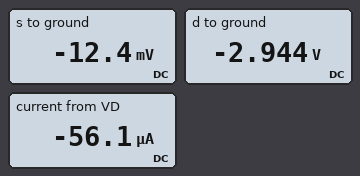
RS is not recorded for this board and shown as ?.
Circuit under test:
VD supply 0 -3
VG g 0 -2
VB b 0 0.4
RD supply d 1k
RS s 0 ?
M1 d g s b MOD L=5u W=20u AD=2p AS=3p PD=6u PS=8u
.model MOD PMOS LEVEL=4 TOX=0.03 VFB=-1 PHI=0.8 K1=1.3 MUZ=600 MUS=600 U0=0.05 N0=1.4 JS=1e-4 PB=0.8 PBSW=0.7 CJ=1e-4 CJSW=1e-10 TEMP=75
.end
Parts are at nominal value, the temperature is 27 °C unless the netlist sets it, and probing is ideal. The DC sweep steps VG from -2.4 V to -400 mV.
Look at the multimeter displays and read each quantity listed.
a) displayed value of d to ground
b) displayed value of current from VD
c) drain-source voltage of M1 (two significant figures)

-2.944 V
-56.1 µA
-2.9 V
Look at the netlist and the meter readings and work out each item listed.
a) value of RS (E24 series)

220 Ω
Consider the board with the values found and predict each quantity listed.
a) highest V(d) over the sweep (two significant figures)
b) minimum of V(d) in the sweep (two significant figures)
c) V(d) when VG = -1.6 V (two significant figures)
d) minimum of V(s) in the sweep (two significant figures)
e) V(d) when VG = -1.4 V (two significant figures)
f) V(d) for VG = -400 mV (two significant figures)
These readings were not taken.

-2.9 V
-3.0 V
-3.0 V
-27 mV
-3.0 V
-3.0 V
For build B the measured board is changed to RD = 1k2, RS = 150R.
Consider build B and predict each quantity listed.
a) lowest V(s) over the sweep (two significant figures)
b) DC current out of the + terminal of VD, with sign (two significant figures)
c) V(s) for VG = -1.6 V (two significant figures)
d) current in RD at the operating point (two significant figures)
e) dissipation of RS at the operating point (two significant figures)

-19 mV
-57 µA
-2.2 mV
57 µA
490 nW
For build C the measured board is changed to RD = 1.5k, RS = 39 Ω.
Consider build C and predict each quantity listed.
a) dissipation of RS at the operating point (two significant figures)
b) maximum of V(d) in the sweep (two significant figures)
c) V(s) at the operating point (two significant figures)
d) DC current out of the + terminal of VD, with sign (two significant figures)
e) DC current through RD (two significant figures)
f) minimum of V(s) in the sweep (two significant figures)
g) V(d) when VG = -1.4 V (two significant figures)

130 nW
-2.8 V
-2.3 mV
-58 µA
58 µA
-5.1 mV
-3.0 V
